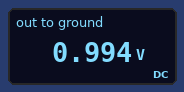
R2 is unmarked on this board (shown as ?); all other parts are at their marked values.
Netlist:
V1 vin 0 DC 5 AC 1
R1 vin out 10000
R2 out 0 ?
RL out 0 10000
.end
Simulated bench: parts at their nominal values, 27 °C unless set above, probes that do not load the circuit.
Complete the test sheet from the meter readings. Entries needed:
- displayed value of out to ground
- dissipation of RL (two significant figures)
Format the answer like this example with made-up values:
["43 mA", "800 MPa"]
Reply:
["0.994 V", "99 µW"]
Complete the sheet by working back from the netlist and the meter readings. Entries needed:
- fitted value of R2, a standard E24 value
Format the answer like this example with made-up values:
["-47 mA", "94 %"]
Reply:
["3.3 kΩ"]
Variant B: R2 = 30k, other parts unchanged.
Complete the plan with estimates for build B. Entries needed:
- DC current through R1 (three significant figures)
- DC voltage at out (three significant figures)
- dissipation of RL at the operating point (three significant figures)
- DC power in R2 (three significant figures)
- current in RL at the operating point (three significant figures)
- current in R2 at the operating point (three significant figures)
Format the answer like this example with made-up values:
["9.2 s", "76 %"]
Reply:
["286 µA", "2.14 V", "459 µW", "153 µW", "214 µA", "71.4 µA"]
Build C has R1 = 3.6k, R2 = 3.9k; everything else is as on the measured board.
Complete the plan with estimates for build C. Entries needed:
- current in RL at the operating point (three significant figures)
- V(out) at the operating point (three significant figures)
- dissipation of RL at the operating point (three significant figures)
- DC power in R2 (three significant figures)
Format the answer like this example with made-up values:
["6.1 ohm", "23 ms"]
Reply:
["219 µA", "2.19 V", "480 µW", "1.23 mW"]
